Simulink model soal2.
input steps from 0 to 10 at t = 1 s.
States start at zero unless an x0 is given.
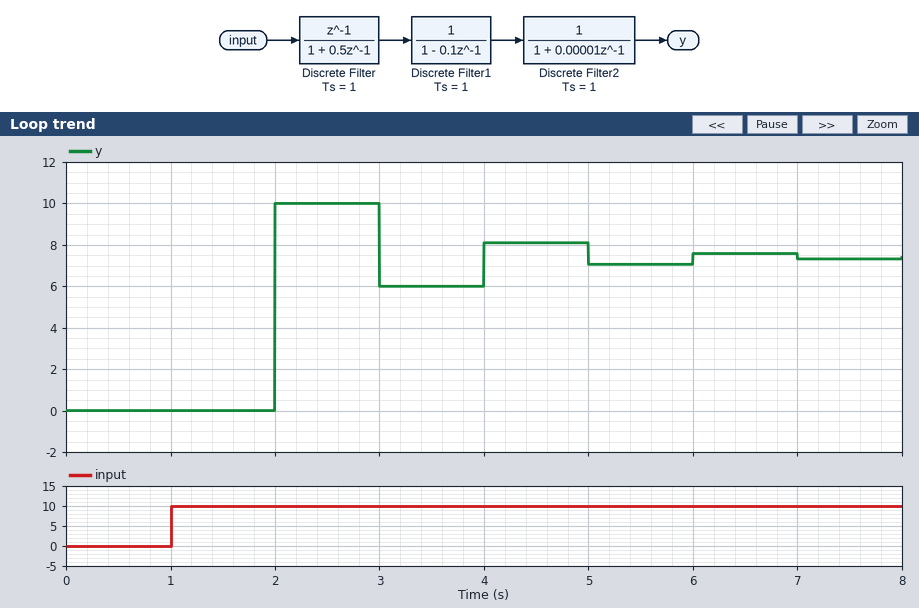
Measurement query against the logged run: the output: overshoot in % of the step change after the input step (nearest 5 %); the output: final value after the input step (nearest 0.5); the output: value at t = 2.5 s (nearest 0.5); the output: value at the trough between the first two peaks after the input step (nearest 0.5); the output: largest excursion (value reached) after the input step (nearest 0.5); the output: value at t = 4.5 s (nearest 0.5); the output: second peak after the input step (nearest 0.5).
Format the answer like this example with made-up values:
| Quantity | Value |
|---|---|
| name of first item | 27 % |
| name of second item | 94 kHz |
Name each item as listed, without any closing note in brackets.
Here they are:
| Quantity | Value |
|---|---|
| the output: overshoot in % of the step change after the input step | 35 % |
| the output: final value after the input step | 7.5 |
| the output: value at t = 2.5 s | 10.0 |
| the output: value at the trough between the first two peaks after the input step | 6.0 |
| the output: largest excursion (value reached) after the input step | 10.0 |
| the output: value at t = 4.5 s | 8.0 |
| the output: second peak after the input step | 8.0 |
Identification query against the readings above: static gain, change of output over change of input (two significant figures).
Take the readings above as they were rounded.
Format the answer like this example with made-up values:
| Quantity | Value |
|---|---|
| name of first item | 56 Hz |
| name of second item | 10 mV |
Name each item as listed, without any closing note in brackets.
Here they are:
| Quantity | Value |
|---|---|
| static gain, change of output over change of input | 0.75 |
